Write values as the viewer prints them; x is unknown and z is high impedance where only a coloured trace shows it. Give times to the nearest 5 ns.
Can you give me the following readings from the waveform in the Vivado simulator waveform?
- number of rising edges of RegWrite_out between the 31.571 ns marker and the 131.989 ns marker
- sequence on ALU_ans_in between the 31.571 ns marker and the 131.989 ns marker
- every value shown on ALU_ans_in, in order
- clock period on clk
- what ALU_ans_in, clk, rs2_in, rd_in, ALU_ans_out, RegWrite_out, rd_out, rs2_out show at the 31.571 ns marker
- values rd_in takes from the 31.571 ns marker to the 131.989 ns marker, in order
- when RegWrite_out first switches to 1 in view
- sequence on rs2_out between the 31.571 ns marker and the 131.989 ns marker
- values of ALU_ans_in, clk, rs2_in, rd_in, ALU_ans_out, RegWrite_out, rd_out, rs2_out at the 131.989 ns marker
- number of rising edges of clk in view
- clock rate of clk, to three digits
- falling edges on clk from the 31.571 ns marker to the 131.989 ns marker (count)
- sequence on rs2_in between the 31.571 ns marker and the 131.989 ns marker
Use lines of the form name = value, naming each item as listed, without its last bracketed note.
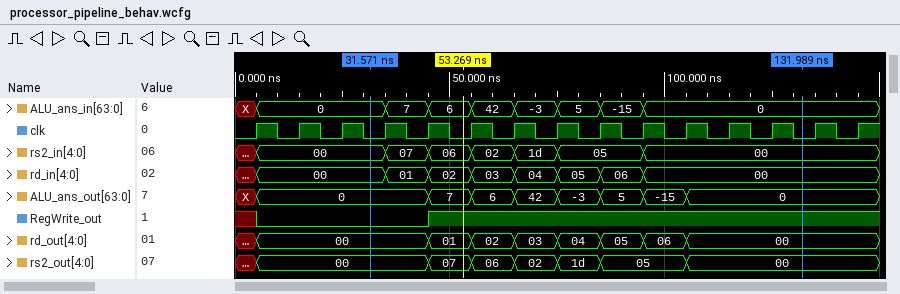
number of rising edges of RegWrite_out between the 31.571 ns marker and the 131.989 ns marker = 1
sequence on ALU_ans_in between the 31.571 ns marker and the 131.989 ns marker = 0, 7, 6, 42, -3, 5, -15, 0
every value shown on ALU_ans_in, in order = X, 0, 7, 6, 42, -3, 5, -15, 0
clock period on clk = 10 ns
what ALU_ans_in, clk, rs2_in, rd_in, ALU_ans_out, RegWrite_out, rd_out, rs2_out show at the 31.571 ns marker = ALU_ans_in=0, clk=0, rs2_in=00, rd_in=00, ALU_ans_out=0, RegWrite_out=0, rd_out=00, rs2_out=00
values rd_in takes from the 31.571 ns marker to the 131.989 ns marker, in order = 00, 01, 02, 03, 04, 05, 06, 00
when RegWrite_out first switches to 1 in view = 45 ns
sequence on rs2_out between the 31.571 ns marker and the 131.989 ns marker = 00, 07, 06, 02, 1d, 05, 00
values of ALU_ans_in, clk, rs2_in, rd_in, ALU_ans_out, RegWrite_out, rd_out, rs2_out at the 131.989 ns marker = ALU_ans_in=0, clk=0, rs2_in=00, rd_in=00, ALU_ans_out=0, RegWrite_out=1, rd_out=00, rs2_out=00
number of rising edges of clk in view = 15
clock rate of clk, to three digits = 100 MHz
falling edges on clk from the 31.571 ns marker to the 131.989 ns marker = 10
sequence on rs2_in between the 31.571 ns marker and the 131.989 ns marker = 00, 07, 06, 02, 1d, 05, 00
